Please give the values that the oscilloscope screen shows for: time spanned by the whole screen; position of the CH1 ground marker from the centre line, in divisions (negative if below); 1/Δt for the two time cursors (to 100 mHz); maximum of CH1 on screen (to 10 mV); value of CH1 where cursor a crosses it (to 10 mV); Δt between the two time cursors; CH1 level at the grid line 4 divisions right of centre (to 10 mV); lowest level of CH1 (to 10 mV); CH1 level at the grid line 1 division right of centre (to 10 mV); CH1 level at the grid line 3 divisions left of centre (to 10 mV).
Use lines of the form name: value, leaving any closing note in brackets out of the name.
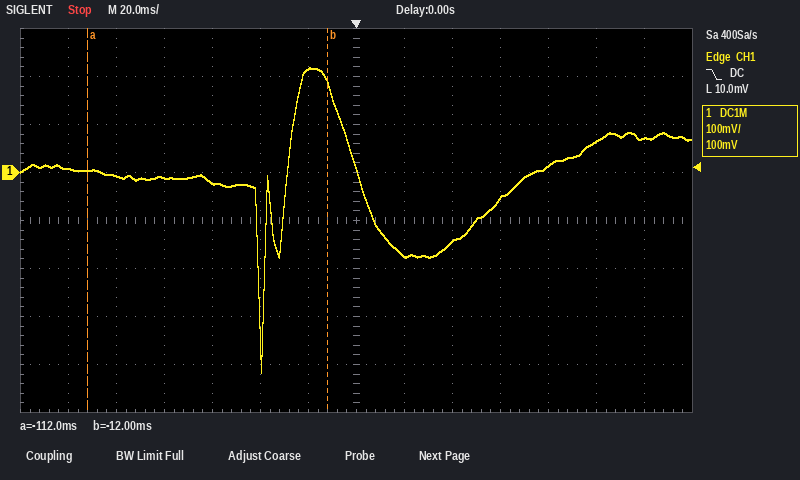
time spanned by the whole screen: 280 ms
position of the CH1 ground marker from the centre line, in divisions: +1.0 div
1/Δt for the two time cursors: 10.0 Hz
maximum of CH1 on screen: 220 mV
value of CH1 where cursor a crosses it: 0 mV
Δt between the two time cursors: 100 ms
CH1 level at the grid line 4 divisions right of centre: 10 mV
lowest level of CH1: -420 mV
CH1 level at the grid line 1 division right of centre: -170 mV
CH1 level at the grid line 3 divisions left of centre: -20 mV
